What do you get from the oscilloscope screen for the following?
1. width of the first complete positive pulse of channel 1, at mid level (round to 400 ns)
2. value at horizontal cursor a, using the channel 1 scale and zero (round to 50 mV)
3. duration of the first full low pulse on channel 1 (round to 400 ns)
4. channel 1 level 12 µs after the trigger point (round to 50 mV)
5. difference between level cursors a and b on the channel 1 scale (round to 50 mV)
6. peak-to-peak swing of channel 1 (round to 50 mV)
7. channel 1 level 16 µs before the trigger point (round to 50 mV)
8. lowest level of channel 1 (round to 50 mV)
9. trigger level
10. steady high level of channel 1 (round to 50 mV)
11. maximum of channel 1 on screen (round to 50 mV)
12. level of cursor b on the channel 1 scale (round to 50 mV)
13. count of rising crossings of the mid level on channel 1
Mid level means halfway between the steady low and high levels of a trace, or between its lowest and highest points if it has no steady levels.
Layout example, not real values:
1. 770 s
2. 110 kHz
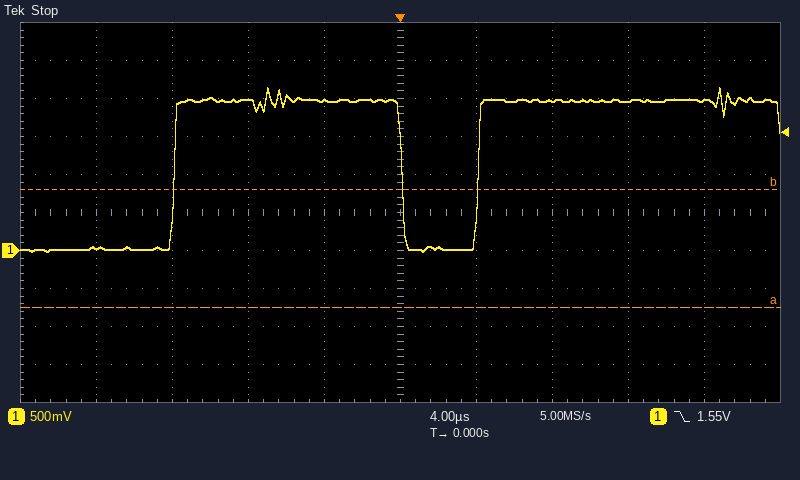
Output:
1. 12.0 µs
2. -750 mV
3. 4.0 µs
4. 1.95 V
5. 1.55 V
6. 2.15 V
7. 50 mV
8. 0 mV
9. 1.55 V
10. 2.00 V
11. 2.15 V
12. 800 mV
13. 2
